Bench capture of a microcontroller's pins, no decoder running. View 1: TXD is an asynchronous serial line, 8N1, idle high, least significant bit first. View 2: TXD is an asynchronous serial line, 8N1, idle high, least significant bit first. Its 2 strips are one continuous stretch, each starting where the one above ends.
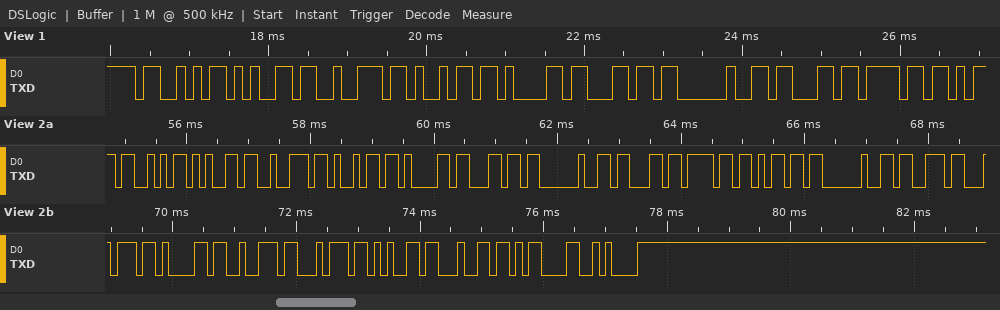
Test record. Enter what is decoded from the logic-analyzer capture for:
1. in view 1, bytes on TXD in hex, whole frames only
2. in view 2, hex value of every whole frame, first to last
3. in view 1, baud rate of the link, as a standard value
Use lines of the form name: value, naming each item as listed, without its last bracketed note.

in view 1, bytes on TXD in hex, whole frames only: 53 65 72 69 61 6C 20 63 6F
in view 2, hex value of every whole frame, first to last: 0x53 0x65 0x72 0x69 0x61 0x6C 0x20 0x63 0x6F 0x6D 0x20 0x73 0x74 0x61 0x72 0x74 0x65 0x64 0x0D 0x0A
in view 1, baud rate of the link, as a standard value: 9600 baud
